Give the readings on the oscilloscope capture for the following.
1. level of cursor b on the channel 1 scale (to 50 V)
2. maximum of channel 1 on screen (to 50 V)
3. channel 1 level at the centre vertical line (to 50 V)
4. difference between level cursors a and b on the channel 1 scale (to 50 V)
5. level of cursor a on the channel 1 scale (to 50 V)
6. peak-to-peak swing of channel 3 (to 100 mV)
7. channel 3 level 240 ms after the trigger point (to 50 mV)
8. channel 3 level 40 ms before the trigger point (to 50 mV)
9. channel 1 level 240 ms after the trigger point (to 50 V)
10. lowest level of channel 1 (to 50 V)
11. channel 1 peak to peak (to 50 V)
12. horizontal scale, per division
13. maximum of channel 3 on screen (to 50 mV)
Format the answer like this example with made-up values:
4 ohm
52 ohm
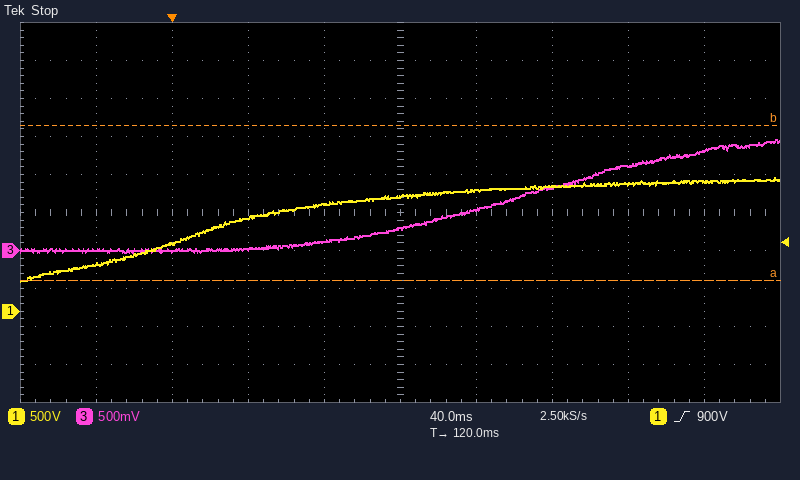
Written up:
2.45 kV
1.75 kV
1.50 kV
2.05 kV
400 V
1.50 V
1.10 V
0 mV
1.70 kV
400 V
1.35 kV
40 ms
1.45 V
